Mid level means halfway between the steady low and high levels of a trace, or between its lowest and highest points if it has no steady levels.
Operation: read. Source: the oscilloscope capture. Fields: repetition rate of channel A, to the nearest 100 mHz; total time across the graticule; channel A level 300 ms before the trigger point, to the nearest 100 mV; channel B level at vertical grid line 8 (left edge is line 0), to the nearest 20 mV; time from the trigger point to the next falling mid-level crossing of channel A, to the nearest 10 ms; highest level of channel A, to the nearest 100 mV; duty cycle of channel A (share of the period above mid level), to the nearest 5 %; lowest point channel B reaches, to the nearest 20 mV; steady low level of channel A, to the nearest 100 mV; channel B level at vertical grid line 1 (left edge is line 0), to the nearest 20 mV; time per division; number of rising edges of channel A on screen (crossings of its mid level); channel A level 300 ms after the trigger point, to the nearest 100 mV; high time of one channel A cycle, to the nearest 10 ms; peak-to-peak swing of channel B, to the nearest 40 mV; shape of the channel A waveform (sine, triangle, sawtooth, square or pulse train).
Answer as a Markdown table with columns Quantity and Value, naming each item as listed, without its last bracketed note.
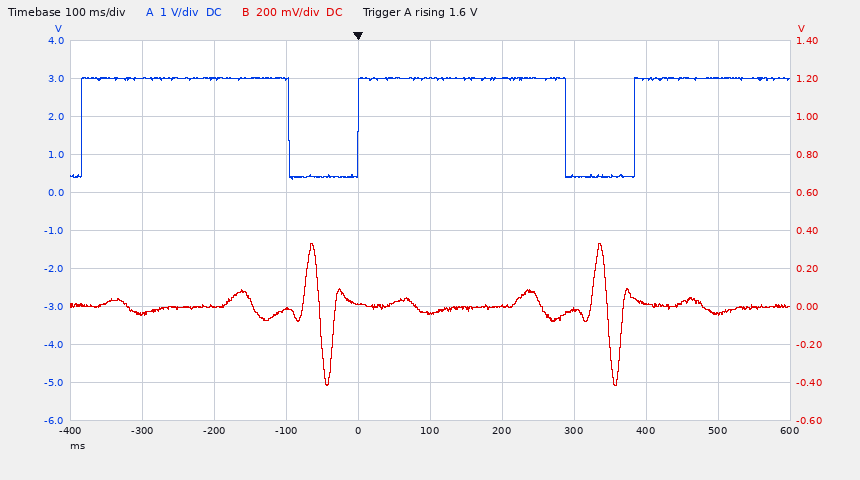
| Quantity | Value |
|---|---|
| repetition rate of channel A, to the nearest 100 mHz | 2.6 Hz |
| total time across the graticule | 1 s |
| channel A level 300 ms before the trigger point, to the nearest 100 mV | 3.0 V |
| channel B level at vertical grid line 8 (left edge is line 0), to the nearest 20 mV | 20 mV |
| time from the trigger point to the next falling mid-level crossing of channel A, to the nearest 10 ms | 290 ms |
| highest level of channel A, to the nearest 100 mV | 3.0 V |
| duty cycle of channel A (share of the period above mid level), to the nearest 5 % | 75 % |
| lowest point channel B reaches, to the nearest 20 mV | -420 mV |
| steady low level of channel A, to the nearest 100 mV | 400 mV |
| channel B level at vertical grid line 1 (left edge is line 0), to the nearest 20 mV | -40 mV |
| time per division | 100 ms |
| number of rising edges of channel A on screen | 3 |
| channel A level 300 ms after the trigger point, to the nearest 100 mV | 400 mV |
| high time of one channel A cycle, to the nearest 10 ms | 290 ms |
| peak-to-peak swing of channel B, to the nearest 40 mV | 760 mV |
| shape of the channel A waveform | pulse train |
